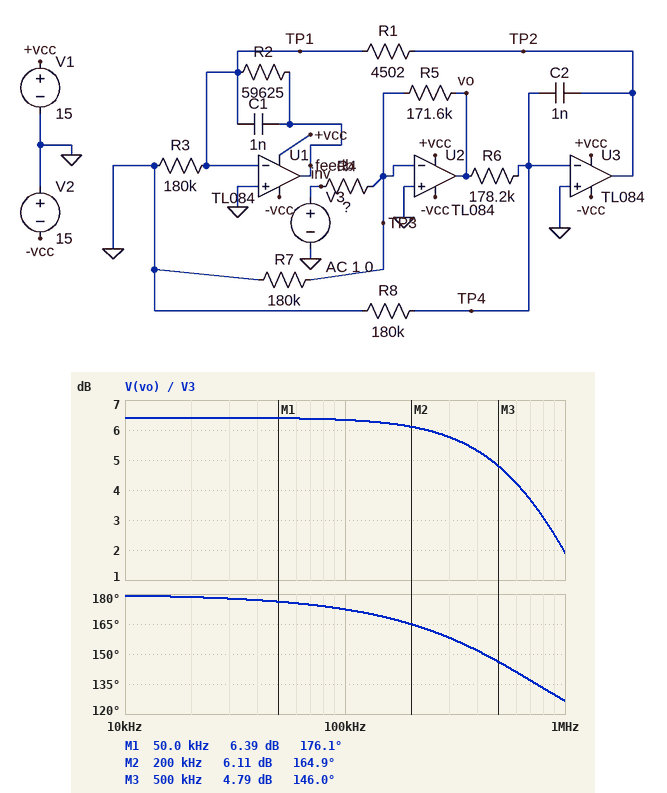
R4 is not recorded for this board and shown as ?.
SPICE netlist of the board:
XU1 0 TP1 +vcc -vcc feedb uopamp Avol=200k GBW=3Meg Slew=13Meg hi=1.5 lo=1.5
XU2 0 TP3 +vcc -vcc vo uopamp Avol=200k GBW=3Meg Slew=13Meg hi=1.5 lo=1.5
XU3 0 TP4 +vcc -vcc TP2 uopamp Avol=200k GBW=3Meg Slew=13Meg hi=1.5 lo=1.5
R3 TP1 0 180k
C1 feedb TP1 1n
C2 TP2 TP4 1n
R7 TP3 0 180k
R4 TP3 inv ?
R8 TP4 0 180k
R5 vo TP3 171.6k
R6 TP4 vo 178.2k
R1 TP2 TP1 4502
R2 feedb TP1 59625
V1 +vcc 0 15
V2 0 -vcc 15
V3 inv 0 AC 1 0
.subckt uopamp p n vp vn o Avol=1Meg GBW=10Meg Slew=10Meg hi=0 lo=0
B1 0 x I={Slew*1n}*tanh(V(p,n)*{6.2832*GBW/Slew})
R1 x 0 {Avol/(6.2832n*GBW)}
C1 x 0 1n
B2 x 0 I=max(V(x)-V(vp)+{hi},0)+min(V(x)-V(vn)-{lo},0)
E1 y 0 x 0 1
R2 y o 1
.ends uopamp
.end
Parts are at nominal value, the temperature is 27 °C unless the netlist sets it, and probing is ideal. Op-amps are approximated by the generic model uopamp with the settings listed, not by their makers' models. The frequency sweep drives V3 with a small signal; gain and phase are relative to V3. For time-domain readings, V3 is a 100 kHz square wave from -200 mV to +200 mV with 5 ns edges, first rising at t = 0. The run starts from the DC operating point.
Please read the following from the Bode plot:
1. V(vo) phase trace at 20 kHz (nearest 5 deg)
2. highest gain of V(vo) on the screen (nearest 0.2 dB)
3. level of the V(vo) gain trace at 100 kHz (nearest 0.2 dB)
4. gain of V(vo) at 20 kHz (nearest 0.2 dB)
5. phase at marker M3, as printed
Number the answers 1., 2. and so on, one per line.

1. 180 deg
2. 6.4 dB
3. 6.4 dB
4. 6.4 dB
5. 146.0 deg
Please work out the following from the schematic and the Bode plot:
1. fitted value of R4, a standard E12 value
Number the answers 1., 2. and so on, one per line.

1. 82 kΩ
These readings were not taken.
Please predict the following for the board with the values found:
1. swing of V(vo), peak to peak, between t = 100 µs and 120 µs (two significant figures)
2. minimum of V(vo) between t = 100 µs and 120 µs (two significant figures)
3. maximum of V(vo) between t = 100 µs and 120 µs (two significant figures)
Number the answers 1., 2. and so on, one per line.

1. 840 mV
2. -420 mV
3. 420 mV
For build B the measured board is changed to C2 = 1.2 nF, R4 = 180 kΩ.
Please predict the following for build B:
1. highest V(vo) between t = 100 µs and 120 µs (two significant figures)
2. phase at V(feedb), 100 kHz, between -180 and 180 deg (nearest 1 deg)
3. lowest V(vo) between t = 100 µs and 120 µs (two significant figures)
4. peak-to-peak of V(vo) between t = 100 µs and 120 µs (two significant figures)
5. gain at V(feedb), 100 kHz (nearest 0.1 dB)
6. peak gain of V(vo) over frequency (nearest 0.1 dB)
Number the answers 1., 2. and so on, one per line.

1. 190 mV
2. -8 deg
3. -190 mV
4. 380 mV
5. -52.2 dB
6. -0.4 dB
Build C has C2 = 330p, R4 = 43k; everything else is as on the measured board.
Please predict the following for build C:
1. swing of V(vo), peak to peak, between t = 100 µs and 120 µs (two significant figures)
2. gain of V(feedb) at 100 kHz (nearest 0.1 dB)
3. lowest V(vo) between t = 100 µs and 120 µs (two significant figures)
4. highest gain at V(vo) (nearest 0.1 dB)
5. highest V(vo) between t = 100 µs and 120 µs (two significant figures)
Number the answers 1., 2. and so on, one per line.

1. 1.6 V
2. -28.7 dB
3. -800 mV
4. 12.0 dB
5. 800 mV
